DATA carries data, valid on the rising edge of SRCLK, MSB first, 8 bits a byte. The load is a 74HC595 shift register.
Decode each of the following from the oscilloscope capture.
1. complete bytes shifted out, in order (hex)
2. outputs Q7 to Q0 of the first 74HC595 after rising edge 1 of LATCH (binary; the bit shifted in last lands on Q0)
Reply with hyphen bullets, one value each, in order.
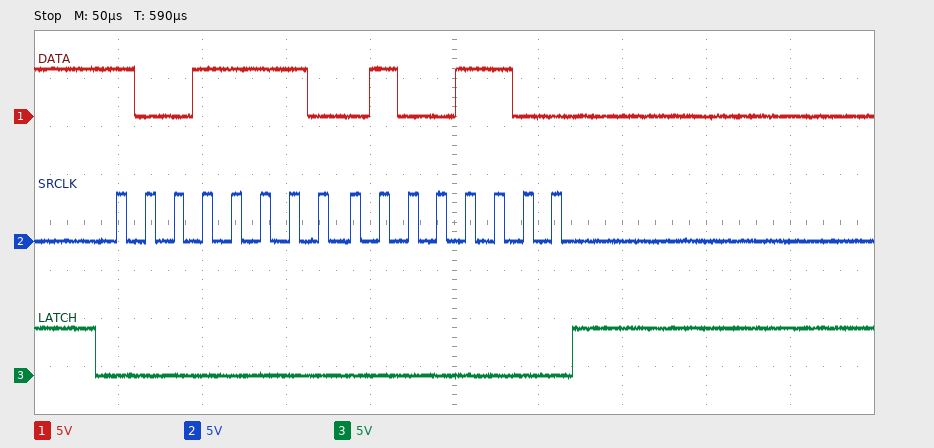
- 9E 4C
- 01001100
